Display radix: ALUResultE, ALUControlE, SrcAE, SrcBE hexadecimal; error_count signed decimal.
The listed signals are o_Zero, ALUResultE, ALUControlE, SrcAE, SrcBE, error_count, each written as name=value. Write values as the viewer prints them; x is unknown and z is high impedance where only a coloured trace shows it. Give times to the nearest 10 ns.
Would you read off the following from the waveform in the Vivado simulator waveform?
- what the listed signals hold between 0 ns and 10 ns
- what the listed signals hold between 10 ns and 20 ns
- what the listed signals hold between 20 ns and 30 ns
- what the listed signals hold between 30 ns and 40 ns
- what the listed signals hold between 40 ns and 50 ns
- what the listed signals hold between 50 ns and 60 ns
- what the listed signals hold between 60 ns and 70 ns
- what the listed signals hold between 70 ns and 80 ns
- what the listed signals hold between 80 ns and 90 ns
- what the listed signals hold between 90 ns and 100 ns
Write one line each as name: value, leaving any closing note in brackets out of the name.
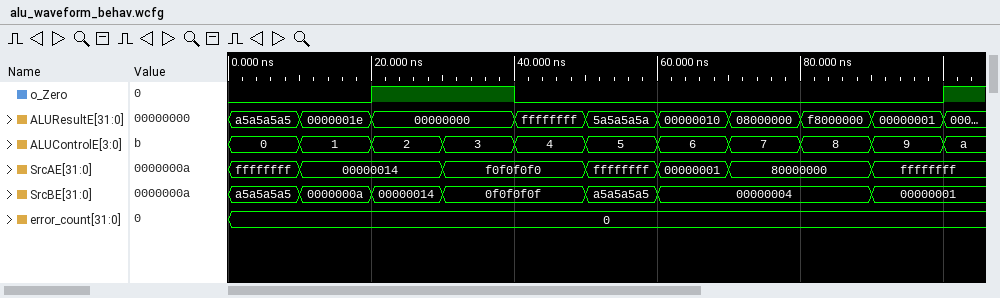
what the listed signals hold between 0 ns and 10 ns: o_Zero=0, ALUResultE=a5a5a5a5, ALUControlE=0, SrcAE=ffffffff, SrcBE=a5a5a5a5, error_count=0
what the listed signals hold between 10 ns and 20 ns: o_Zero=0, ALUResultE=0000001e, ALUControlE=1, SrcAE=00000014, SrcBE=0000000a, error_count=0
what the listed signals hold between 20 ns and 30 ns: o_Zero=1, ALUResultE=00000000, ALUControlE=2, SrcAE=00000014, SrcBE=00000014, error_count=0
what the listed signals hold between 30 ns and 40 ns: o_Zero=1, ALUResultE=00000000, ALUControlE=3, SrcAE=f0f0f0f0, SrcBE=0f0f0f0f, error_count=0
what the listed signals hold between 40 ns and 50 ns: o_Zero=0, ALUResultE=ffffffff, ALUControlE=4, SrcAE=f0f0f0f0, SrcBE=0f0f0f0f, error_count=0
what the listed signals hold between 50 ns and 60 ns: o_Zero=0, ALUResultE=5a5a5a5a, ALUControlE=5, SrcAE=ffffffff, SrcBE=a5a5a5a5, error_count=0
what the listed signals hold between 60 ns and 70 ns: o_Zero=0, ALUResultE=00000010, ALUControlE=6, SrcAE=00000001, SrcBE=00000004, error_count=0
what the listed signals hold between 70 ns and 80 ns: o_Zero=0, ALUResultE=08000000, ALUControlE=7, SrcAE=80000000, SrcBE=00000004, error_count=0
what the listed signals hold between 80 ns and 90 ns: o_Zero=0, ALUResultE=f8000000, ALUControlE=8, SrcAE=80000000, SrcBE=00000004, error_count=0
what the listed signals hold between 90 ns and 100 ns: o_Zero=0, ALUResultE=00000001, ALUControlE=9, SrcAE=ffffffff, SrcBE=00000001, error_count=0
